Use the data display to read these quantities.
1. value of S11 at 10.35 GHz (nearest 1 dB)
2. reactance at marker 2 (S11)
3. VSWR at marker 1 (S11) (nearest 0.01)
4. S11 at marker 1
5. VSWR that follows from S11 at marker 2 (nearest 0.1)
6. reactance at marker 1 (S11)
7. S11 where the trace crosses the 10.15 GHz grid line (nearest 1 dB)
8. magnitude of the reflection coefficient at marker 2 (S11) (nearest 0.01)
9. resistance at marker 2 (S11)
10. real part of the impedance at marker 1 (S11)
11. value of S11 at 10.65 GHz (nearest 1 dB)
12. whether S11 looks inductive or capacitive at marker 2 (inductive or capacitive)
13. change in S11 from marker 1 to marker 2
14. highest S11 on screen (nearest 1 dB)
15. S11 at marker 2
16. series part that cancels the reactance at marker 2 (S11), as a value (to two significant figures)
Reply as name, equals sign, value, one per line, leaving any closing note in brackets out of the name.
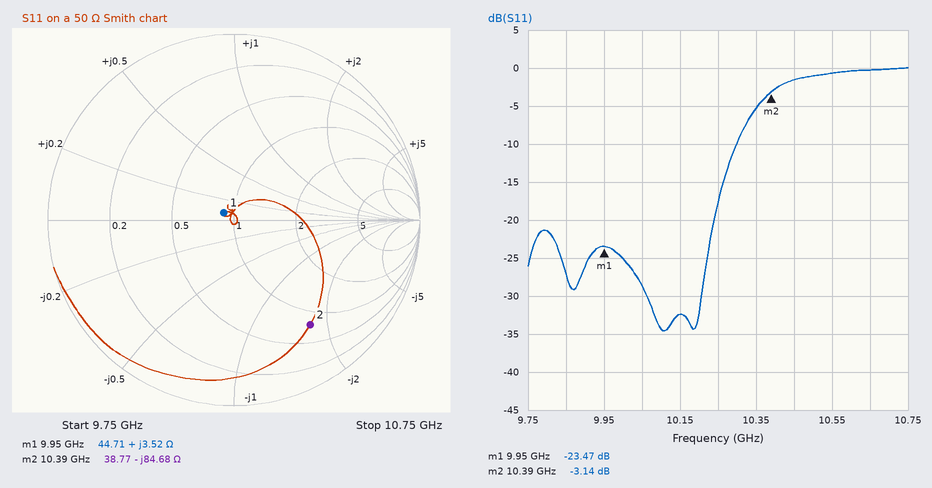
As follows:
value of S11 at 10.35 GHz = -5 dB
reactance at marker 2 = -84.68 Ω
VSWR at marker 1 (S11) = 1.14
S11 at marker 1 = -23.47 dB
VSWR that follows from S11 at marker 2 = 5.6
reactance at marker 1 = +3.52 Ω
S11 where the trace crosses the 10.15 GHz grid line = -32 dB
magnitude of the reflection coefficient at marker 2 (S11) = 0.70
resistance at marker 2 = 38.77 Ω
real part of the impedance at marker 1 = 44.71 Ω
value of S11 at 10.65 GHz = 0 dB
whether S11 looks inductive or capacitive at marker 2 = capacitive
change in S11 from marker 1 to marker 2 = 20.33 dB
highest S11 on screen = 0 dB
S11 at marker 2 = -3.14 dB
series part that cancels the reactance at marker 2 (S11), as a value = 1.3 nH
